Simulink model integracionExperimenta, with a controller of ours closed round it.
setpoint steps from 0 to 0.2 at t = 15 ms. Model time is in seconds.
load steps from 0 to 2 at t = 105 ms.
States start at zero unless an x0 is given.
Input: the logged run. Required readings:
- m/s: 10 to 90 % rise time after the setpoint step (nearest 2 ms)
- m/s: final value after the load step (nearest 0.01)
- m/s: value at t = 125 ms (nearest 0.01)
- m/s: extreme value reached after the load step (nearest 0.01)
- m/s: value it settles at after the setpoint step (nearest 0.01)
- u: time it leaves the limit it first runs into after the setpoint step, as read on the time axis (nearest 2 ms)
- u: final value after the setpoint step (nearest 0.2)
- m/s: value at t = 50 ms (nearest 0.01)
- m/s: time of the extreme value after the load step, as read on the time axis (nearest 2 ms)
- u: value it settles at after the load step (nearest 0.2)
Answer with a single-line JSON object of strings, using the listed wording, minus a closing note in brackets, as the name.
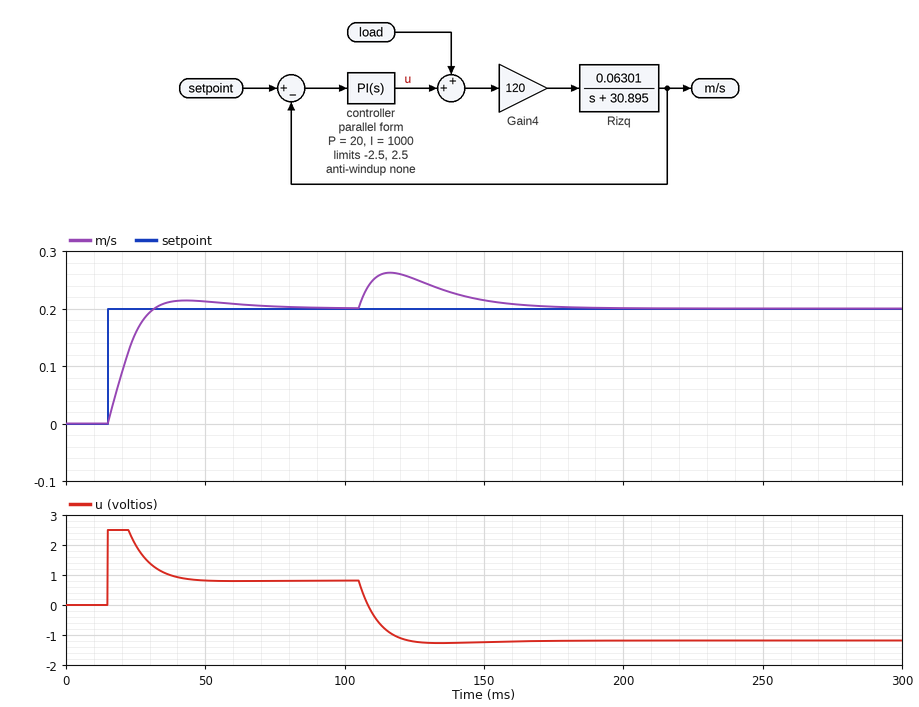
{"m/s: 10 to 90 % rise time after the setpoint step": "12 ms", "m/s: final value after the load step": "0.20", "m/s: value at t = 125 ms": "0.25", "m/s: extreme value reached after the load step": "0.26", "m/s: value it settles at after the setpoint step": "0.20", "u: time it leaves the limit it first runs into after the setpoint step, as read on the time axis": "22 ms", "u: final value after the setpoint step": "0.8", "m/s: value at t = 50 ms": "0.21", "m/s: time of the extreme value after the load step, as read on the time axis": "116 ms", "u: value it settles at after the load step": "-1.2"}
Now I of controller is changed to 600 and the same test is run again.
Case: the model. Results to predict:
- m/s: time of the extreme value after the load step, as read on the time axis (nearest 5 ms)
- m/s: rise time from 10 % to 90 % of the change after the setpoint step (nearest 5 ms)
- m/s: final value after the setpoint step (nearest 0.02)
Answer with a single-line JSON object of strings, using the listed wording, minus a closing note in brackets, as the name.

{"m/s: time of the extreme value after the load step, as read on the time axis": "120 ms", "m/s: rise time from 10 % to 90 % of the change after the setpoint step": "15 ms", "m/s: final value after the setpoint step": "0.20"}
